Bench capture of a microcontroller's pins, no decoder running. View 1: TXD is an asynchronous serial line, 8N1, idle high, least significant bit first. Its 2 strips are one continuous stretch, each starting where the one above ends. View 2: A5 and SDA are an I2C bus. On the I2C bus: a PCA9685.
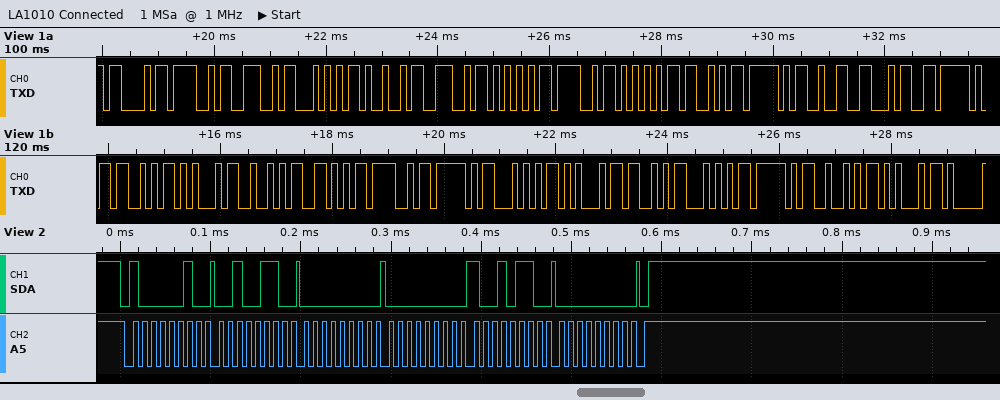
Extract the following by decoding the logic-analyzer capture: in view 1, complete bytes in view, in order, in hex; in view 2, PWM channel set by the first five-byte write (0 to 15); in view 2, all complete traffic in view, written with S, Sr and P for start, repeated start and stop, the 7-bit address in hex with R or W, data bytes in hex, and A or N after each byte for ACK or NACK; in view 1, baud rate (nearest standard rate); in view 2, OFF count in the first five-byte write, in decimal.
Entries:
43 4F 4E 54 49 4E 55 4F 55 53 5F 32 34 5F 53 45 52 56 4F 5F 54 45 53 54 5F 52 45
8
S 41W A 26 A 00 A 00 A 96 A 00 A P
9600 baud
150
